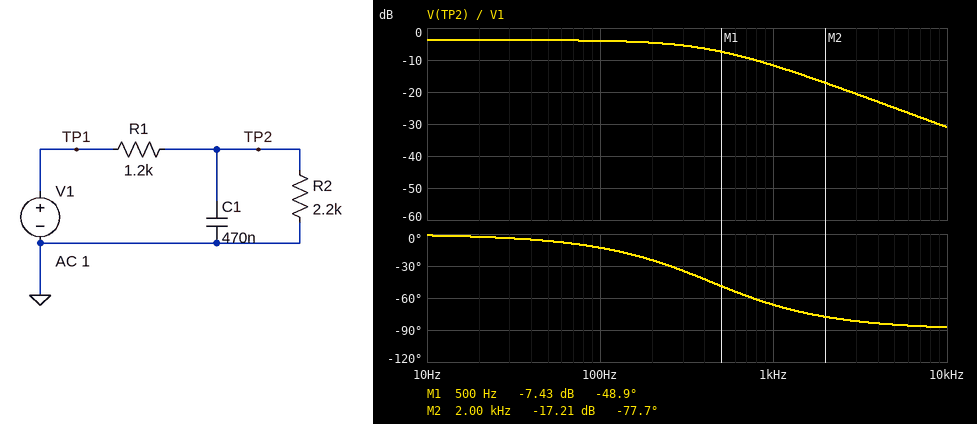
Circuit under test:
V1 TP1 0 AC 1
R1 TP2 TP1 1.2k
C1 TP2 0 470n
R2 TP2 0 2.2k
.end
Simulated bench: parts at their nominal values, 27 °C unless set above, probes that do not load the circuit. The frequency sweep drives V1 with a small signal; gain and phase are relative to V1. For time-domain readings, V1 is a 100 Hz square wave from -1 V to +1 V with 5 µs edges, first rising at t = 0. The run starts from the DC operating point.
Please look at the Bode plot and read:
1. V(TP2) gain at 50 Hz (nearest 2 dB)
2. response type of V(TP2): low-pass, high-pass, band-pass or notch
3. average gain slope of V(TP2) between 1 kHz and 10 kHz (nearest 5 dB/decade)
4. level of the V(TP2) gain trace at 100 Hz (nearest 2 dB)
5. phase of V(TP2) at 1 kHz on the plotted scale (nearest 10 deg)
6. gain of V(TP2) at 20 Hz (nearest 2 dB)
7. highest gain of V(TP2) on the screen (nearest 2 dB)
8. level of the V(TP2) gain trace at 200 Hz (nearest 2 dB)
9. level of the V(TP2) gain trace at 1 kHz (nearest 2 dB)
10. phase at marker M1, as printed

-4 dB
low-pass
-20 dB/decade
-4 dB
-70 deg
-4 dB
-4 dB
-4 dB
-12 dB
-48.9 deg
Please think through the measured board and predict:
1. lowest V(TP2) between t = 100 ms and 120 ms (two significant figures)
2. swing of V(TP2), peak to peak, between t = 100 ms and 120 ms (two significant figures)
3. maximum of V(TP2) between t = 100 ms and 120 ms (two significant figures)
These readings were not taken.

-650 mV
1.3 V
650 mV
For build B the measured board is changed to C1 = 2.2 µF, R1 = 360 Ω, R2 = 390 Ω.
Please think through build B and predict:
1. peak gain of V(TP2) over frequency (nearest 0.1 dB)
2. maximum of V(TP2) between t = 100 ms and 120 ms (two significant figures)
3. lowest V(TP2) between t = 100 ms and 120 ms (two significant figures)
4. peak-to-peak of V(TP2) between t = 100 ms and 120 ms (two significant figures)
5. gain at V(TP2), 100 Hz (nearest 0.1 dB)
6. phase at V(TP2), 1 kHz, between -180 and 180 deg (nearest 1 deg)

-5.7 dB
520 mV
-520 mV
1.0 V
-6.0 dB
-69 deg
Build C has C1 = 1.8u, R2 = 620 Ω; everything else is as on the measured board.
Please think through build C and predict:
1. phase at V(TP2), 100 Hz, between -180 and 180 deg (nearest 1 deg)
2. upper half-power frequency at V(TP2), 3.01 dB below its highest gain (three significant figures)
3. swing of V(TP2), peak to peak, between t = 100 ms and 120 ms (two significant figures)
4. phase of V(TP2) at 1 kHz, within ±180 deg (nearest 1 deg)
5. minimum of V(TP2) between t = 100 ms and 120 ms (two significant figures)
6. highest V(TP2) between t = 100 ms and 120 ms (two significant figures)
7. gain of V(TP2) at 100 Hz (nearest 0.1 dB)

-25 deg
216 Hz
680 mV
-78 deg
-340 mV
340 mV
-10.2 dB
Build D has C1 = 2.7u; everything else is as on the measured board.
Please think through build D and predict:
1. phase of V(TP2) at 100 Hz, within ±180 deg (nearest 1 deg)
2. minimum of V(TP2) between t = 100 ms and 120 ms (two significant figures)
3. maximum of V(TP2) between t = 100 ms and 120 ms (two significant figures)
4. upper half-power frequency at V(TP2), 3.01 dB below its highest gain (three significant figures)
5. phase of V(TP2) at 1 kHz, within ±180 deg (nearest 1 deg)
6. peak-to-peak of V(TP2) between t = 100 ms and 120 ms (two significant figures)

-53 deg
-540 mV
540 mV
75.9 Hz
-86 deg
1.1 V
